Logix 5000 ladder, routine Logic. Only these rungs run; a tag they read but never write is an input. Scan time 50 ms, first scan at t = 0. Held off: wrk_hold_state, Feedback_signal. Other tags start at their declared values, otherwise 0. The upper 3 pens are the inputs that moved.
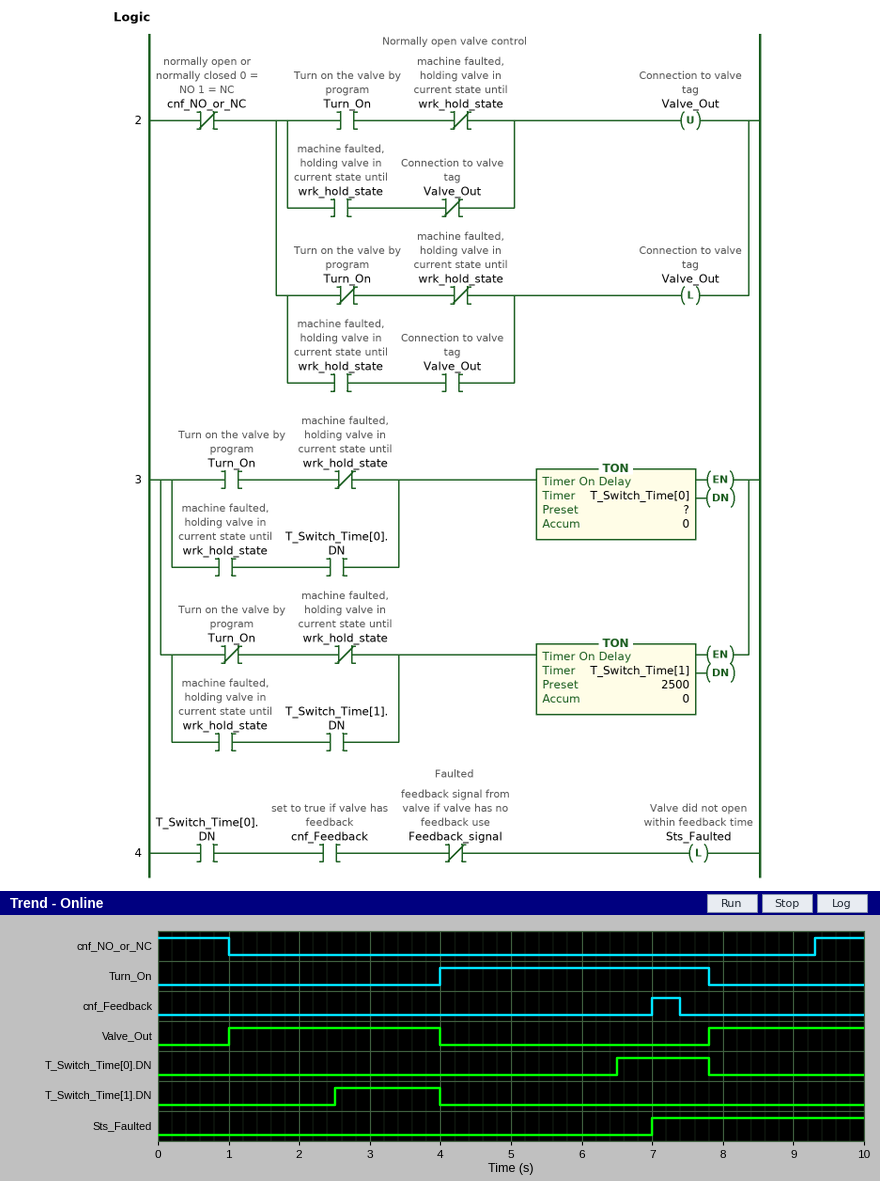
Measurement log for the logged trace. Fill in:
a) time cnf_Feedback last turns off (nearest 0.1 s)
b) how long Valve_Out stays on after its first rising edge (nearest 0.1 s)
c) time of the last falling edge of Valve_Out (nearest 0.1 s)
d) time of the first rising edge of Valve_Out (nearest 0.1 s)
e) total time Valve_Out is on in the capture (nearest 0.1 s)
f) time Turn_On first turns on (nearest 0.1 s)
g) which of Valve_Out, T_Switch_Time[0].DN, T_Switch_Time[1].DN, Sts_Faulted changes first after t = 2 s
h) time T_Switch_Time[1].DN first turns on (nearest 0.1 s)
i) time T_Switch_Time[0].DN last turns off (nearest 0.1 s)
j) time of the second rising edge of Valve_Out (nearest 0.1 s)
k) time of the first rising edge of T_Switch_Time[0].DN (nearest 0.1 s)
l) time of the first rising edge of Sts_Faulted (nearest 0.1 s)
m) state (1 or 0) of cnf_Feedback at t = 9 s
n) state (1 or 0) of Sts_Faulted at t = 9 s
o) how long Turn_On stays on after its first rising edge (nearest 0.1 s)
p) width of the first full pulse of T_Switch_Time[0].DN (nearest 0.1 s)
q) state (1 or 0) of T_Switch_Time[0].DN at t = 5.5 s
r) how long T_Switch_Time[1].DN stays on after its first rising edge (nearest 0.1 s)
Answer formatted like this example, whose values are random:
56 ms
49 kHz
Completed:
7.4 s
3.0 s
4.0 s
1.0 s
5.2 s
4.0 s
T_Switch_Time[1].DN
2.5 s
7.8 s
7.8 s
6.5 s
7.0 s
0
1
3.8 s
1.3 s
0
1.5 s
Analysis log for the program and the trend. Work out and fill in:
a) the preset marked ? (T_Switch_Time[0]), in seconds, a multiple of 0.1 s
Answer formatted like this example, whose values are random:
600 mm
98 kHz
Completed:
2.5 s
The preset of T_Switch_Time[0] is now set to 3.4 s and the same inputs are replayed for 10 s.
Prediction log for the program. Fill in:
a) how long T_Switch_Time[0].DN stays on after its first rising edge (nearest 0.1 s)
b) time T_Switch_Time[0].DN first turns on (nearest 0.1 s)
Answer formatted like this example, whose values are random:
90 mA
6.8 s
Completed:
0.4 s
7.4 s
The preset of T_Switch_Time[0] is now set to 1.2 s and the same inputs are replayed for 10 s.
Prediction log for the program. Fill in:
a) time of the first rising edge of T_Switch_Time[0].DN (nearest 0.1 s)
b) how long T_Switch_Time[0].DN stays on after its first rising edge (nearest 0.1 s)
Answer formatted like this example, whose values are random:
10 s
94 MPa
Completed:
5.2 s
2.6 s
